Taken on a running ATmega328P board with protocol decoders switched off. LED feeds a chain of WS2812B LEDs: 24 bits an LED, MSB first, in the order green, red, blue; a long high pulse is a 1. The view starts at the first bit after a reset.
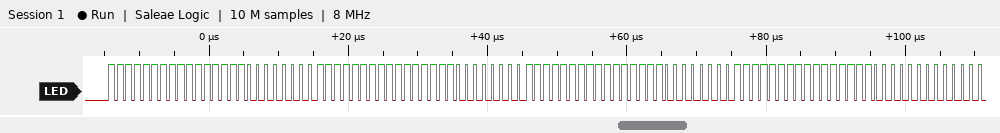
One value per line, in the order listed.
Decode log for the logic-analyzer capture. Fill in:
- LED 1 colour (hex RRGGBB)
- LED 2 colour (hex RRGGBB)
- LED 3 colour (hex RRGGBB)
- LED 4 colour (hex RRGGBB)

#FFFF00
#FFFF00
#FFFF00
#FFFF00
